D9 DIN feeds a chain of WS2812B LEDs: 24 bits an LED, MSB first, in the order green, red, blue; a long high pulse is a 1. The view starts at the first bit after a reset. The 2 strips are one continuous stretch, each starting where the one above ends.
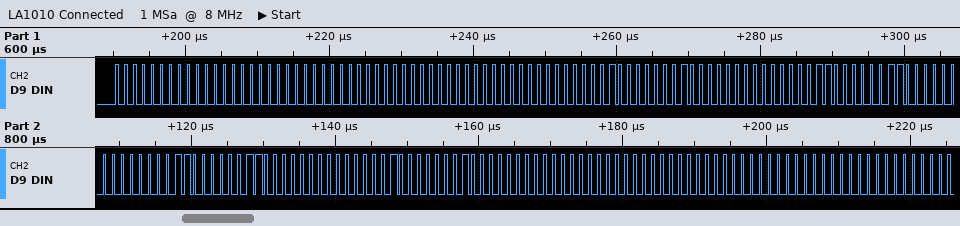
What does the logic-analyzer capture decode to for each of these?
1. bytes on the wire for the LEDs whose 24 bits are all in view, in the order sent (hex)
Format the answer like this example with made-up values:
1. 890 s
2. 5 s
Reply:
1. 00 00 00 00 00 00 01 01 00 03 03 00 03 03 00 02 02 00 00 00 00
